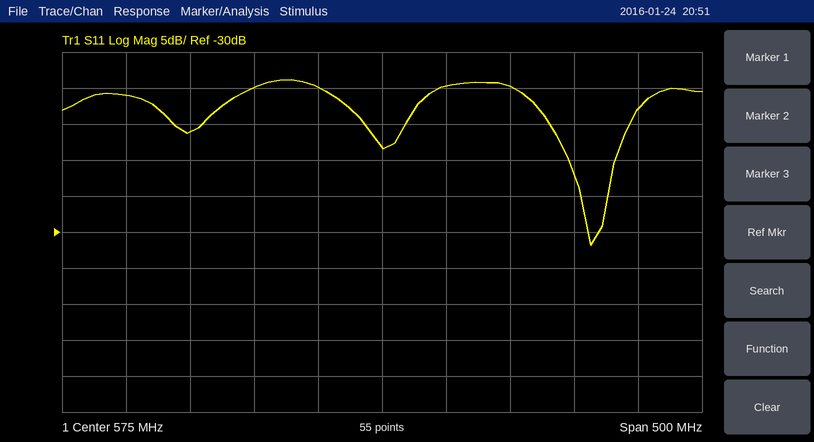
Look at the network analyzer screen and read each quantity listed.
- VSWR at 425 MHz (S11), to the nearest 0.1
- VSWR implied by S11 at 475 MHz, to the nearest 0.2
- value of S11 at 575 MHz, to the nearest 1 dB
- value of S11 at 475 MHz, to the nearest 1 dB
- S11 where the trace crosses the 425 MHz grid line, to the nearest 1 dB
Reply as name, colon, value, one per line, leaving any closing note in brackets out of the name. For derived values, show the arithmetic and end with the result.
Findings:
VSWR at 425 MHz (S11), to the nearest 0.1: |Γ| = 10^(-16/20) = 0.1585; VSWR = (1 + 0.1585)/(1 − 0.1585) ≈ 1.4
VSWR implied by S11 at 475 MHz, to the nearest 0.2: |Γ| = 10^(-10/20) = 0.3162; VSWR = (1 + 0.3162)/(1 − 0.3162) ≈ 1.92, so 2.0 to the nearest 0.2
value of S11 at 575 MHz, to the nearest 1 dB: -18 dB
value of S11 at 475 MHz, to the nearest 1 dB: -10 dB
S11 where the trace crosses the 425 MHz grid line, to the nearest 1 dB: -16 dB
